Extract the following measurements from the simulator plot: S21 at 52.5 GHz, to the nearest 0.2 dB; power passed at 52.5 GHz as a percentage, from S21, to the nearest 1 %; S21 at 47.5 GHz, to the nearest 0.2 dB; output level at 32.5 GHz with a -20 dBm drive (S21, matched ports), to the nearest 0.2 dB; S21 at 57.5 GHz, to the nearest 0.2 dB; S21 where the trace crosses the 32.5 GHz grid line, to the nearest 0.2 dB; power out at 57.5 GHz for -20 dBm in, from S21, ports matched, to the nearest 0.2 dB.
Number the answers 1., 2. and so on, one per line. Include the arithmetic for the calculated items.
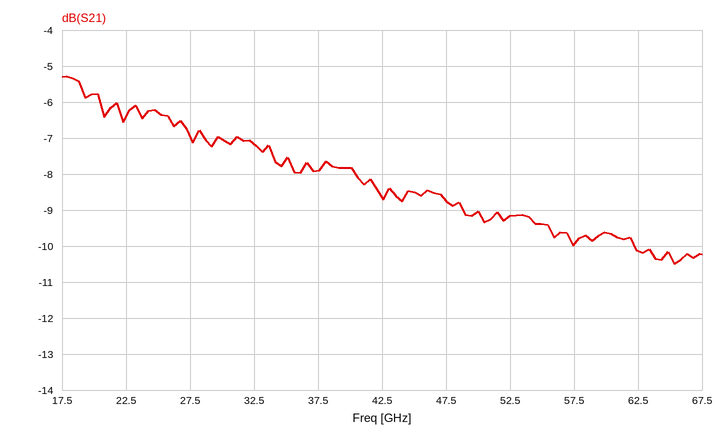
1. -9.2 dB
2. 10^(-9.2/10) ≈ 12 %
3. -8.8 dB
4. -20 dBm + (-7.2 dB) = -27.2 dBm
5. -10.0 dB
6. -7.2 dB
7. -20 dBm + (-10.0 dB) = -30.0 dBm
